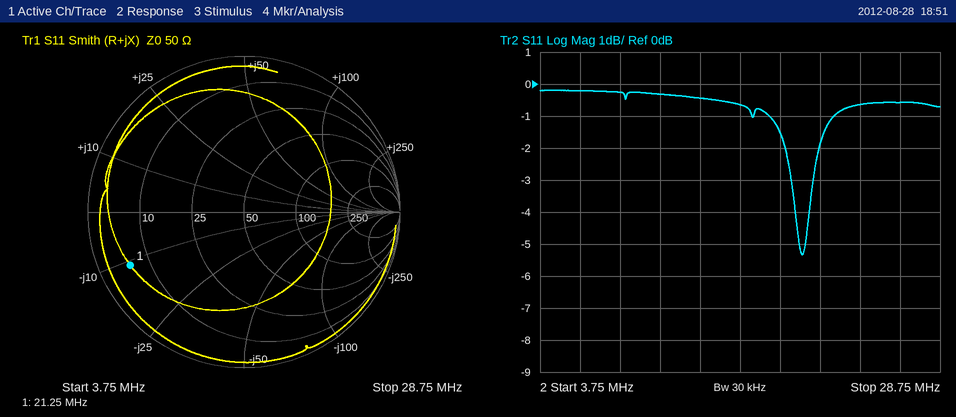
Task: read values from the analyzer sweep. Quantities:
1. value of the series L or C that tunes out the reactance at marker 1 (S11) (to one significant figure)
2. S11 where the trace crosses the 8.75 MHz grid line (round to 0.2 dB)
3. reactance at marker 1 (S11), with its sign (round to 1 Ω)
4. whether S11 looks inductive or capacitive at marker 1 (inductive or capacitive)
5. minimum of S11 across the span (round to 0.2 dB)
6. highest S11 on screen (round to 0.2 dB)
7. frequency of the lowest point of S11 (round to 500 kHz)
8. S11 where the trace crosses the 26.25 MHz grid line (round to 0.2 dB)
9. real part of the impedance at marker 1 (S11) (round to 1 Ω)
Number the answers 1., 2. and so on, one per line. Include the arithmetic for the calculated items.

1. L = 11 Ω/(2π × 21.25 MHz) ≈ 82.4 nH, so 80 nH to one significant figure
2. -0.2 dB
3. -11 Ω
4. capacitive
5. -5.4 dB
6. -0.2 dB
7. 20.0 MHz
8. -0.6 dB
9. 6 Ω
